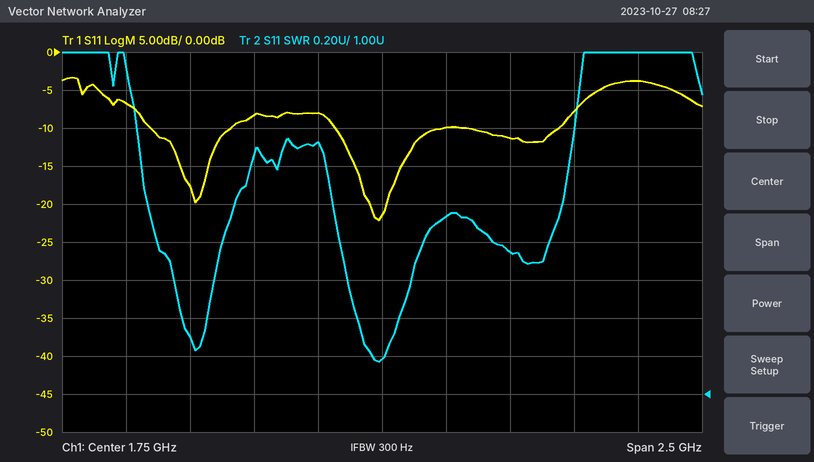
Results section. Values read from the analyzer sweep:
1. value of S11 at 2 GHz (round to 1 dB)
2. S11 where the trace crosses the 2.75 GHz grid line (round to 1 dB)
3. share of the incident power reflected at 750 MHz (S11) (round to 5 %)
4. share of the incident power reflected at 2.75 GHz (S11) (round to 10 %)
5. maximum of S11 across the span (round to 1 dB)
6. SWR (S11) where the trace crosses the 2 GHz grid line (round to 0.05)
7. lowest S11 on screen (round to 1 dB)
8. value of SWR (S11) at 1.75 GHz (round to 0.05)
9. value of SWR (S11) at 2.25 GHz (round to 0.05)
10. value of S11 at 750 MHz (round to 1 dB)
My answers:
-10 dB
-4 dB
20 %
40 %
-3 dB
1.95
-22 dB
1.20
1.75
-7 dB
